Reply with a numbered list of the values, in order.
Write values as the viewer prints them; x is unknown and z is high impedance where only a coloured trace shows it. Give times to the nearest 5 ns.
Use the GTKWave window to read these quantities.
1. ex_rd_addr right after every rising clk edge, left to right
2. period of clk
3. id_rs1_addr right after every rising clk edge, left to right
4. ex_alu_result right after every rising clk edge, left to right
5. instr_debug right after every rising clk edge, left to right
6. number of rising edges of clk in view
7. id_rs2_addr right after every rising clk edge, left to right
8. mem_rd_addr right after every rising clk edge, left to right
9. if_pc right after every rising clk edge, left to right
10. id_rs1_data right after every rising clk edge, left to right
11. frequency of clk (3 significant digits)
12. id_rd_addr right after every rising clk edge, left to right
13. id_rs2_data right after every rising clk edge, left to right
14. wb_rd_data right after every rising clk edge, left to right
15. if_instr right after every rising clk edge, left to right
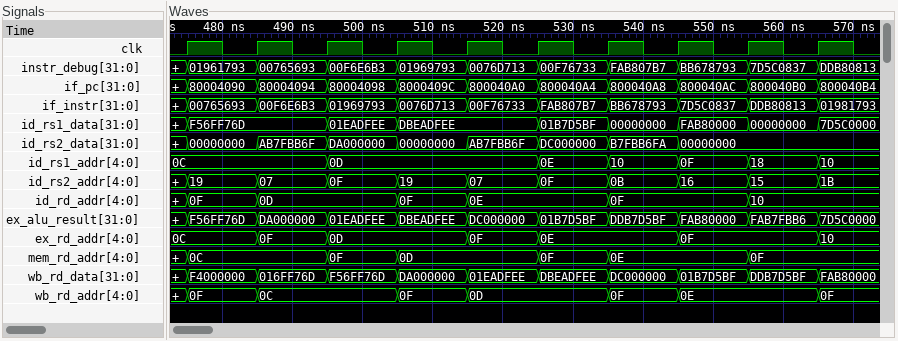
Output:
1. 0C, 0F, 0D, 0D, 0F, 0E, 0E, 0F, 0F, 10
2. 10 ns
3. 0C, 0C, 0D, 0D, 0D, 0E, 10, 0F, 18, 10
4. F56FF76D, DA000000, 01EADFEE, DBEADFEE, DC000000, 01B7D5BF, DDB7D5BF, FAB80000, FAB7FBB6, 7D5C0000
5. 01961793, 00765693, 00F6E6B3, 01969793, 0076D713, 00F76733, FAB807B7, BB678793, 7D5C0837, DDB80813
6. 10
7. 19, 07, 0F, 19, 07, 0F, 0B, 16, 15, 1B
8. 0C, 0C, 0F, 0D, 0D, 0F, 0E, 0E, 0F, 0F
9. 80004090, 80004094, 80004098, 8000409C, 800040A0, 800040A4, 800040A8, 800040AC, 800040B0, 800040B4
10. F56FF76D, F56FF76D, 01EADFEE, DBEADFEE, DBEADFEE, 01B7D5BF, 00000000, FAB80000, 00000000, 7D5C0000
11. 100 MHz
12. 0F, 0D, 0D, 0F, 0E, 0E, 0F, 0F, 10, 10
13. 00000000, AB7FBB6F, DA000000, 00000000, AB7FBB6F, DC000000, B7FBB6FA, 00000000, 00000000, 00000000
14. F4000000, 016FF76D, F56FF76D, DA000000, 01EADFEE, DBEADFEE, DC000000, 01B7D5BF, DDB7D5BF, FAB80000
15. 00765693, 00F6E6B3, 01969793, 0076D713, 00F76733, FAB807B7, BB678793, 7D5C0837, DDB80813, 01981793
